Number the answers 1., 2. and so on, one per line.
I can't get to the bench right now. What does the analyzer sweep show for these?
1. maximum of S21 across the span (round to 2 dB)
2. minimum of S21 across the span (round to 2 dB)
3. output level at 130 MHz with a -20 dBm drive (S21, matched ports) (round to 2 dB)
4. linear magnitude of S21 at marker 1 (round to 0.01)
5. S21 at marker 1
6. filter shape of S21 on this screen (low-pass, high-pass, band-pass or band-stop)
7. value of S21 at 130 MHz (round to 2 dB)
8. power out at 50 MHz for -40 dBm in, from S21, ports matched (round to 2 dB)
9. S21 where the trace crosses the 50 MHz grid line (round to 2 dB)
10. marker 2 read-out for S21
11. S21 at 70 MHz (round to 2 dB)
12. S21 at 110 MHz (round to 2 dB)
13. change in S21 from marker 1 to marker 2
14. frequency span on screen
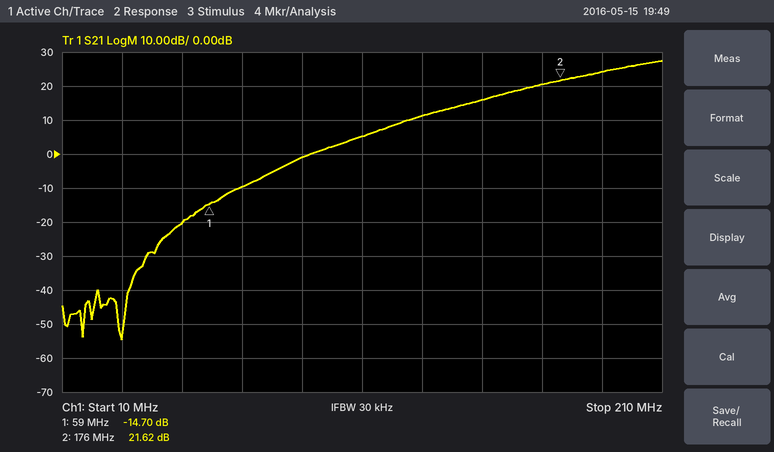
1. 28 dB
2. -54 dB
3. -8 dBm
4. 0.18
5. -14.70 dB
6. high-pass
7. 12 dB
8. -60 dBm
9. -20 dB
10. 21.62 dB
11. -10 dB
12. 6 dB
13. 36.32 dB
14. 200 MHz
